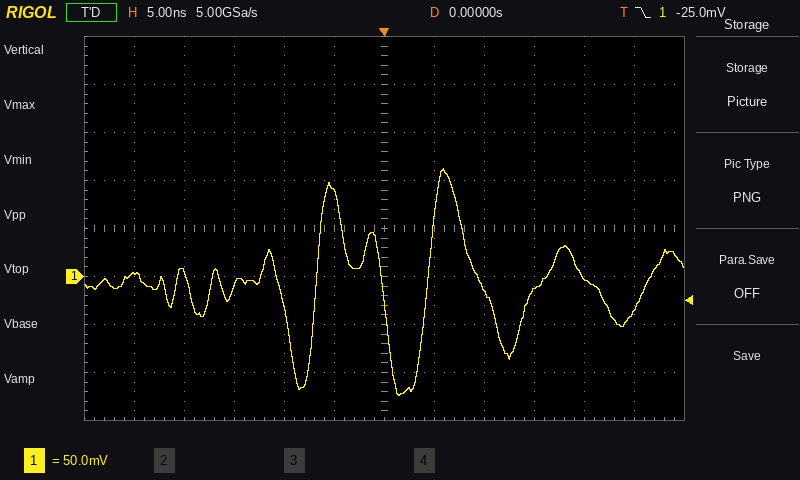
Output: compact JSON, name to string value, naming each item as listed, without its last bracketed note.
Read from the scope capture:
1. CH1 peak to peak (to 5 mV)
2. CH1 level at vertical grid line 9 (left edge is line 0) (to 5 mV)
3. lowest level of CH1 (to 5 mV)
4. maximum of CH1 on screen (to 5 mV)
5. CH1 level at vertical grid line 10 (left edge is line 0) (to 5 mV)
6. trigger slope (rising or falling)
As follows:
{"CH1 peak to peak": "235 mV", "CH1 level at vertical grid line 9 (left edge is line 0)": "-15 mV", "lowest level of CH1": "-125 mV", "maximum of CH1 on screen": "110 mV", "CH1 level at vertical grid line 10 (left edge is line 0)": "0 mV", "trigger slope": "falling"}
